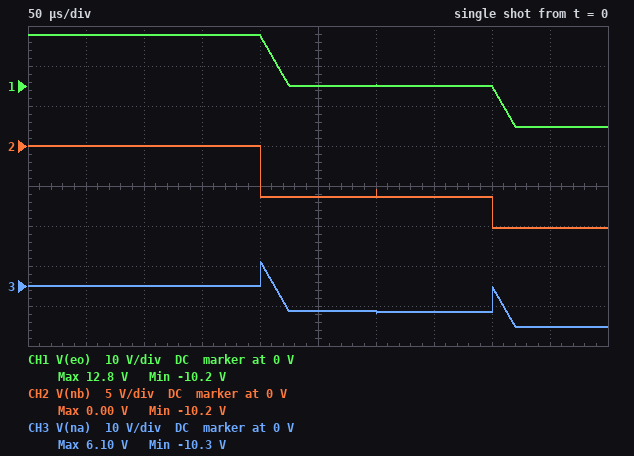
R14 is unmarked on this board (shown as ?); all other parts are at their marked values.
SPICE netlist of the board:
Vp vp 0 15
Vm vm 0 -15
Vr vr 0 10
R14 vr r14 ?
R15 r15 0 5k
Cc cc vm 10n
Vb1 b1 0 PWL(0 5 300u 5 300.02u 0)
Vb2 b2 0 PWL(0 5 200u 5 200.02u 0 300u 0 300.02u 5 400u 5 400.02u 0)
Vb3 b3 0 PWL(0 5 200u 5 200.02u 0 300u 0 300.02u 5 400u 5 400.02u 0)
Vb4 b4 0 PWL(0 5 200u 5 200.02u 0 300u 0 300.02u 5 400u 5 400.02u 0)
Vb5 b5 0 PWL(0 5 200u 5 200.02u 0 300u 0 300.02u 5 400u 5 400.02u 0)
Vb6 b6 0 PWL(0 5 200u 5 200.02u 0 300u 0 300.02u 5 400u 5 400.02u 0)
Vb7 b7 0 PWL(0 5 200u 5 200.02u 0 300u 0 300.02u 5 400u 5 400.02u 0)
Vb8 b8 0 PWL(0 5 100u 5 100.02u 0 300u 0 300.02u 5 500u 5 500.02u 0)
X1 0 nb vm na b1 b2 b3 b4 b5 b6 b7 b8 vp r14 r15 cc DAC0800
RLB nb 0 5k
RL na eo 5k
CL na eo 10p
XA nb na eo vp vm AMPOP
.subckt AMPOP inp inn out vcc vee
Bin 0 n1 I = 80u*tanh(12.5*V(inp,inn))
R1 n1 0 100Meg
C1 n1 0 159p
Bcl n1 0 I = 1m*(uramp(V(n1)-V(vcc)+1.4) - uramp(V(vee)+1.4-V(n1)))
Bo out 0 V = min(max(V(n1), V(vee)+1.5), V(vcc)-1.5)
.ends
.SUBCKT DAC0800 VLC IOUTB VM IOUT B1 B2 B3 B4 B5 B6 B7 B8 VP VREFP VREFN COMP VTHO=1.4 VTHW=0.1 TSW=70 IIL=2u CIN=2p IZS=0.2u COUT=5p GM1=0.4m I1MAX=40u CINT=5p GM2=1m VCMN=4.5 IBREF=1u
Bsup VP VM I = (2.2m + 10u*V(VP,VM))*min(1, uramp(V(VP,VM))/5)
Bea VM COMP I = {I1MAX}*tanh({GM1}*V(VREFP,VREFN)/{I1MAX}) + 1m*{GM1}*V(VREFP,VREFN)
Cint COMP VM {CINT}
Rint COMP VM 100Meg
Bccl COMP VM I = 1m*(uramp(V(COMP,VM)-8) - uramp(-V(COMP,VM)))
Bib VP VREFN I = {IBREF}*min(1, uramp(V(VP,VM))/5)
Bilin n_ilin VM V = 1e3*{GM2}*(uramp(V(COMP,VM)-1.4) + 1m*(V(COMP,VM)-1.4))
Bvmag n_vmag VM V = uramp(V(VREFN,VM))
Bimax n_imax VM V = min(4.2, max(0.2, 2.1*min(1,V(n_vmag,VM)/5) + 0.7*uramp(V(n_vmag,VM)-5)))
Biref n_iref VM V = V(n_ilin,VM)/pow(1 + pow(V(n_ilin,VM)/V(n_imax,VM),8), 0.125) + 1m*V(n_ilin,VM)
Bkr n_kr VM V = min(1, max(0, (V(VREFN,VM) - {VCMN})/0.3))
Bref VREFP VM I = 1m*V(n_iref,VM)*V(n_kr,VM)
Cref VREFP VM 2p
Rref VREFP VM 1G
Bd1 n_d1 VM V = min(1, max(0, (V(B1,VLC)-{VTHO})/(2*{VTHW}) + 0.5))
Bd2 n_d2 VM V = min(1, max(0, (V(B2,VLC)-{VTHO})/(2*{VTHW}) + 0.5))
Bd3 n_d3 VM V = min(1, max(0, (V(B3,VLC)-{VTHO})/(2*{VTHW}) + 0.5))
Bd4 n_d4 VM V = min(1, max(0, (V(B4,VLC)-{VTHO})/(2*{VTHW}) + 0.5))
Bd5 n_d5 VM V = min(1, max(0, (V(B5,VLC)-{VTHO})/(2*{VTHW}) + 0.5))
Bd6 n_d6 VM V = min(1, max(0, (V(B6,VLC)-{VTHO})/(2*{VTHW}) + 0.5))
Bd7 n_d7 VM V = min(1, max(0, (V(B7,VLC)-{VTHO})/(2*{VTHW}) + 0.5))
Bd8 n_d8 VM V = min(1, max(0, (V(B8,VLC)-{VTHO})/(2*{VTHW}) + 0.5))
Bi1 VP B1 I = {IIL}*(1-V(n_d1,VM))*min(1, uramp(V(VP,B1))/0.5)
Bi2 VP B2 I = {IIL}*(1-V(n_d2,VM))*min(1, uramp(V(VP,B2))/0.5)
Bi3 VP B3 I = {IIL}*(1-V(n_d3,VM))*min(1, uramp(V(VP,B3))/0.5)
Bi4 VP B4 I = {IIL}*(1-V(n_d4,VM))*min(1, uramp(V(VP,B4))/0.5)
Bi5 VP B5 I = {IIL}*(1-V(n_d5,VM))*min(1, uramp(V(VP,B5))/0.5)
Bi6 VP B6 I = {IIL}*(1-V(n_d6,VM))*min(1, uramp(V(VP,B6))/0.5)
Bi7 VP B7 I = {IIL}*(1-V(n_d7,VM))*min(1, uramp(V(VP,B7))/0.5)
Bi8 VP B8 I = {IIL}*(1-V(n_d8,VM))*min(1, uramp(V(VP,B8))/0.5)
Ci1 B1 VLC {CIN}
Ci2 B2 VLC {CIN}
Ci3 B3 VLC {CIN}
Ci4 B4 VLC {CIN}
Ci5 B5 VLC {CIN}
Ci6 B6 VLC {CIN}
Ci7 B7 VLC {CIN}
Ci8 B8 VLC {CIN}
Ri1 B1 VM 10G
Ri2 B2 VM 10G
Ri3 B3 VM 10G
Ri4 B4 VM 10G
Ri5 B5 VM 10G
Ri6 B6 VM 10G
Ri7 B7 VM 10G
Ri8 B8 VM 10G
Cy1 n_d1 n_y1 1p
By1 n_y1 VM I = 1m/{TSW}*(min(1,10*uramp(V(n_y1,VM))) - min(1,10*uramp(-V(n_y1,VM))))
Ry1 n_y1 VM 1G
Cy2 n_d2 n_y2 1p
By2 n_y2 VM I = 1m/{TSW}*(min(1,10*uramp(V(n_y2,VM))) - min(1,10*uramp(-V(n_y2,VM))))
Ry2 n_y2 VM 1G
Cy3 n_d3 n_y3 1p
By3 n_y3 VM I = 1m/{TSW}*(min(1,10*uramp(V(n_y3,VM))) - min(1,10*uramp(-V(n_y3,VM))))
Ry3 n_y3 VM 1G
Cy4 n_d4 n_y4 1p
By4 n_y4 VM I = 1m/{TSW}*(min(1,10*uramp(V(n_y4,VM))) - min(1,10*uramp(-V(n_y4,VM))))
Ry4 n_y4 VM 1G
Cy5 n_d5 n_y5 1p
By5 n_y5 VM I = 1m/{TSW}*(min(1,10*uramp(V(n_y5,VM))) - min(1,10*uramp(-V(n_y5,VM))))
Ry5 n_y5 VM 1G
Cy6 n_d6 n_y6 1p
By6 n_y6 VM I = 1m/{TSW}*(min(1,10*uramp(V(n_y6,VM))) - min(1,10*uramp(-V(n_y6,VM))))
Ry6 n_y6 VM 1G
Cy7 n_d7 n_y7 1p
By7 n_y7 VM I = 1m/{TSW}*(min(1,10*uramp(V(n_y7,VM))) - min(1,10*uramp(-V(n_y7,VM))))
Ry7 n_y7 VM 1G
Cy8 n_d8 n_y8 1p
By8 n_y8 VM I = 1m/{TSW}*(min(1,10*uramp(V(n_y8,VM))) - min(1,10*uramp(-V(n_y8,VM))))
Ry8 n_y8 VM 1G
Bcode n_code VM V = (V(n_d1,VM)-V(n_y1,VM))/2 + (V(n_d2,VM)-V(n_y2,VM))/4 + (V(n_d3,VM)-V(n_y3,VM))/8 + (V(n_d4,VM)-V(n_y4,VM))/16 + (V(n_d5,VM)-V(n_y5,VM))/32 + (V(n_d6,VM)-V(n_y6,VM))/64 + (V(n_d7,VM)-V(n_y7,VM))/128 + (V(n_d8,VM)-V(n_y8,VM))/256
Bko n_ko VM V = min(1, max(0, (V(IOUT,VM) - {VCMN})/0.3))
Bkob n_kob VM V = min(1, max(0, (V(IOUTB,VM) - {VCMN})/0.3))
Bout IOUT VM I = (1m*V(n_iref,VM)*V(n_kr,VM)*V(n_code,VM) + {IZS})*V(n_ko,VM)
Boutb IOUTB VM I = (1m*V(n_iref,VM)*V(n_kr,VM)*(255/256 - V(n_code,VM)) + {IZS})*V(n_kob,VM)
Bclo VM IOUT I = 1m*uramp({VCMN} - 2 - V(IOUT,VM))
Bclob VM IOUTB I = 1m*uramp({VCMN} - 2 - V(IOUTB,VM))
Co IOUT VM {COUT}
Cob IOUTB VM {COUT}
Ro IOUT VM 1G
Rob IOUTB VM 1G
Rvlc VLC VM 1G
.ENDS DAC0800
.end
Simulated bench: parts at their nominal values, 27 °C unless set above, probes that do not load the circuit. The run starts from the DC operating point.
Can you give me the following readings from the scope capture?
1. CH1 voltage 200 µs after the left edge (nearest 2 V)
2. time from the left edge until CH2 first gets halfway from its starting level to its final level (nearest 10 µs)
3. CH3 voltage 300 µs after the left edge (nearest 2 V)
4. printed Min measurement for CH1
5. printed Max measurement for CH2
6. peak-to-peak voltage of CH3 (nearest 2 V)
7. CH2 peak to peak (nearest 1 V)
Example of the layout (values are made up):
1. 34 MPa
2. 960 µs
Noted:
1. 12 V
2. 200 µs
3. -6 V
4. -10.2 V
5. 0.00 V
6. 16 V
7. 10 V
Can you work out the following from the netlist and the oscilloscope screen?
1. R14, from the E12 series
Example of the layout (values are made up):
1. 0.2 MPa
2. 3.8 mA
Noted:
1. 3.9 kΩ
